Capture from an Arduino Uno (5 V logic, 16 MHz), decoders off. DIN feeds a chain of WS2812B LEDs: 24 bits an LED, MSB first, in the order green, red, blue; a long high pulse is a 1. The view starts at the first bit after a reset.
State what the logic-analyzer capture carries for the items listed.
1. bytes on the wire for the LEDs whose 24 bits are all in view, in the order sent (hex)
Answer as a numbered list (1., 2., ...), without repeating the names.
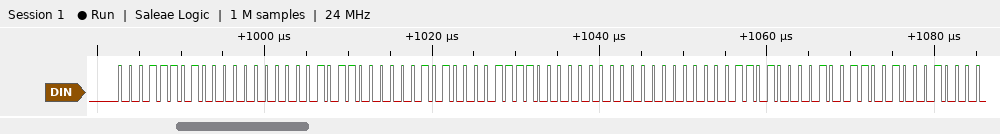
1. 1D 00 16 05 0F 00 00 1A 13
